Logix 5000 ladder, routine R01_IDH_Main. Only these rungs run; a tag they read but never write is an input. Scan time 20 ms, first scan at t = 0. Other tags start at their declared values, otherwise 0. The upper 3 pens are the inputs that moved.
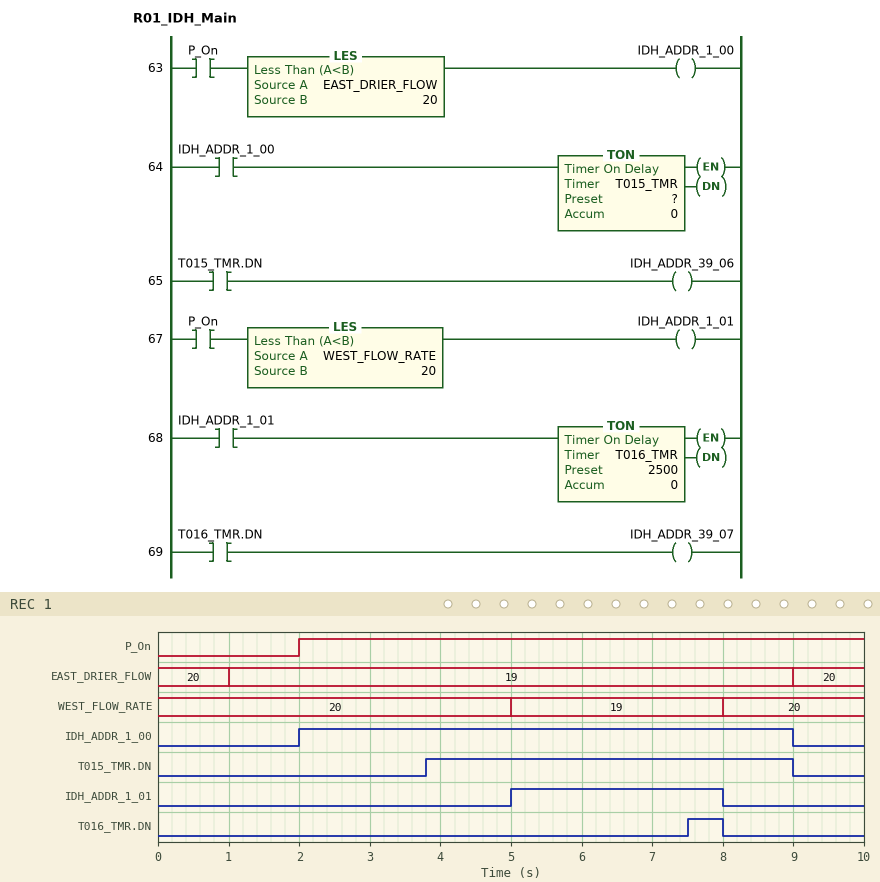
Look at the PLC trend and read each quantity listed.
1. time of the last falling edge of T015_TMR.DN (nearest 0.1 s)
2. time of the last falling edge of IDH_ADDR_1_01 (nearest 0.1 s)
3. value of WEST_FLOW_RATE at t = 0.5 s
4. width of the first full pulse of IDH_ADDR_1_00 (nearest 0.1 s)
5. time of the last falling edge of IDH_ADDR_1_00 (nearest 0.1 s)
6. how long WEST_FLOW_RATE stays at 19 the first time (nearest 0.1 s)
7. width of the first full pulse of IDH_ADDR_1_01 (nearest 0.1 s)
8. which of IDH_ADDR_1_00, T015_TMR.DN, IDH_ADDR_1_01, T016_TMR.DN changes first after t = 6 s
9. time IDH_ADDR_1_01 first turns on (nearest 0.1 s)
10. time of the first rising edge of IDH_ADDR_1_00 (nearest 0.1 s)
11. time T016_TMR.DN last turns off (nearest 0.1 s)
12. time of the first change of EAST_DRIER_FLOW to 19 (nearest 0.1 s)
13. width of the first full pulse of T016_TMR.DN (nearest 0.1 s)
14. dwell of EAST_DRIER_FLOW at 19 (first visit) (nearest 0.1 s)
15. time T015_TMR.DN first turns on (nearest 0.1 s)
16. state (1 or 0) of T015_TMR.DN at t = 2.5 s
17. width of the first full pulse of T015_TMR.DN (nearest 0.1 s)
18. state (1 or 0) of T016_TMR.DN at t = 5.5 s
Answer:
9.0 s
8.0 s
20
7.0 s
9.0 s
3.0 s
3.0 s
T016_TMR.DN
5.0 s
2.0 s
8.0 s
1.0 s
0.5 s
8.0 s
3.8 s
0
5.2 s
0
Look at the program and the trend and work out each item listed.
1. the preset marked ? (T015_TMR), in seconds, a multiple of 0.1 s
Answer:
1.8 s
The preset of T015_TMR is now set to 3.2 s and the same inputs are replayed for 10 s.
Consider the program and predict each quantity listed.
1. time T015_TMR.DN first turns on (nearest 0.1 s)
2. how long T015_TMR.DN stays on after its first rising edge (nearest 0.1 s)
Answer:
5.2 s
3.8 s
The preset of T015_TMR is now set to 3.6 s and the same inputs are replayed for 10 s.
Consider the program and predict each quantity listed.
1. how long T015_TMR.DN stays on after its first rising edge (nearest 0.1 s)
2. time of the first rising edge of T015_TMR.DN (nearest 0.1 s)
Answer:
3.4 s
5.6 s
